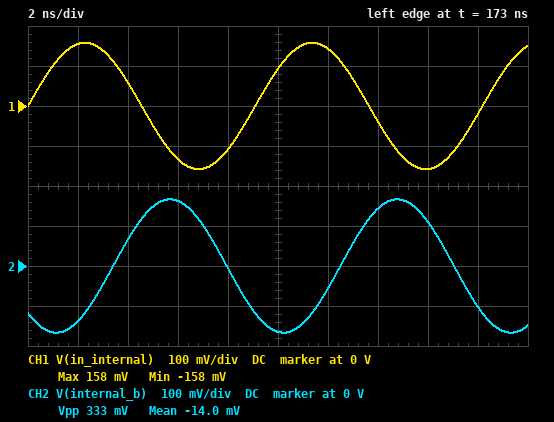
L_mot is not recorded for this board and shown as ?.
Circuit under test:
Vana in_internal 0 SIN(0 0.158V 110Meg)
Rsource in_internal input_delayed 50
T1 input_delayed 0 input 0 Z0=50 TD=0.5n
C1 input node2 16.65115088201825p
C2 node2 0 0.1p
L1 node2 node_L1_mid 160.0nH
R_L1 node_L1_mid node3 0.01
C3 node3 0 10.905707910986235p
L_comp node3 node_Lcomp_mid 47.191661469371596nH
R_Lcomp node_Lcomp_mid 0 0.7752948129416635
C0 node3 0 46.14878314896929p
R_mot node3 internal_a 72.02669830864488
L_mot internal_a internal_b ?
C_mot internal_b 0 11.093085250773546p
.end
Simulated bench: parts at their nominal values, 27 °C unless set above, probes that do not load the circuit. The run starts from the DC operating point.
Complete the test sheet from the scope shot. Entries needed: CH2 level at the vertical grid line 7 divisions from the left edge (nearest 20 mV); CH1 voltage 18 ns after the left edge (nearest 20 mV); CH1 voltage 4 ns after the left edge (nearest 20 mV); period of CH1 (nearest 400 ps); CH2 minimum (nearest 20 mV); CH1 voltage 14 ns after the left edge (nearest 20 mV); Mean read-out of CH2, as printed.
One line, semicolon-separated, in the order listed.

140 mV; -20 mV; 60 mV; 9.2 ns; -160 mV; -40 mV; -14.0 mV
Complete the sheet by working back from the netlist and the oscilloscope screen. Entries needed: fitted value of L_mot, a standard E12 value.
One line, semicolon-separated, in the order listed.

180 nH
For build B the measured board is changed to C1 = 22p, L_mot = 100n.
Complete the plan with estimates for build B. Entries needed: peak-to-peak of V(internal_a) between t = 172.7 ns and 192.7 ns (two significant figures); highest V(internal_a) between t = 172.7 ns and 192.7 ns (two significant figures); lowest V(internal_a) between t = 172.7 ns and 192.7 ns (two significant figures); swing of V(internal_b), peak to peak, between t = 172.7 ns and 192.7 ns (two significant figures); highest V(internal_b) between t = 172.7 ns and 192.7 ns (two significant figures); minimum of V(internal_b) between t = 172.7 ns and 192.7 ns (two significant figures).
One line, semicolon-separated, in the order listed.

150 mV; 74 mV; -74 mV; 310 mV; 160 mV; -160 mV
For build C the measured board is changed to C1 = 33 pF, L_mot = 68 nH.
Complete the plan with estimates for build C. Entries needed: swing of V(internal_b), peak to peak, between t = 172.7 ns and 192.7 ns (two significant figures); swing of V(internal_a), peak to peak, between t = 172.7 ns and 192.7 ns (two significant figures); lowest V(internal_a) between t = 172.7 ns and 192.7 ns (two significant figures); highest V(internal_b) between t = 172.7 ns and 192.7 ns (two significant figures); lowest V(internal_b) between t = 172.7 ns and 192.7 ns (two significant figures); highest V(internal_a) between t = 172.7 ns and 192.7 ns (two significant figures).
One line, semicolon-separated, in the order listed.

300 mV; 190 mV; -95 mV; 150 mV; -150 mV; 95 mV
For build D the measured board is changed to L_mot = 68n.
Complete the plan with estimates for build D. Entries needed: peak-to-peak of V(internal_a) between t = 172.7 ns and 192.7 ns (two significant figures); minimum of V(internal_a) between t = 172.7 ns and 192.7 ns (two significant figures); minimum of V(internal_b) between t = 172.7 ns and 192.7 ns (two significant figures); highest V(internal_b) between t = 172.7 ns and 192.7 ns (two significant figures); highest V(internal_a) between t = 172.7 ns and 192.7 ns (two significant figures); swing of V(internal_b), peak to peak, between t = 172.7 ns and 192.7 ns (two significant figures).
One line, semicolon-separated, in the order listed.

180 mV; -89 mV; -140 mV; 140 mV; 89 mV; 280 mV
